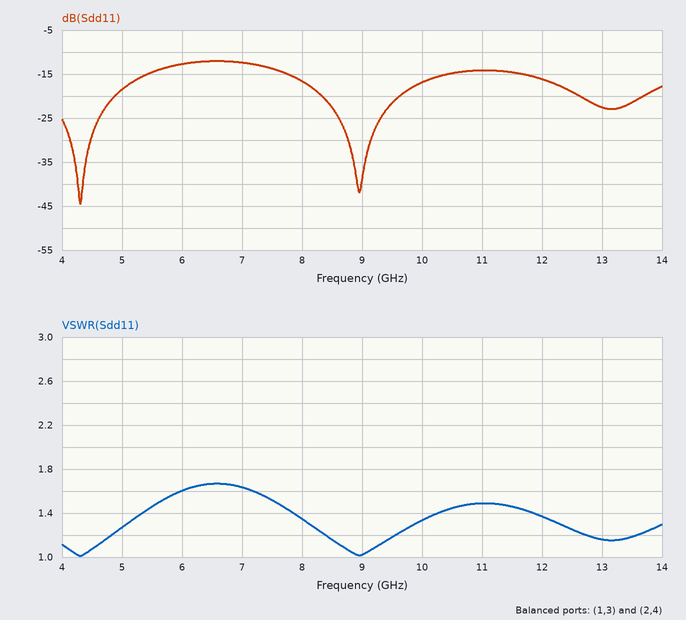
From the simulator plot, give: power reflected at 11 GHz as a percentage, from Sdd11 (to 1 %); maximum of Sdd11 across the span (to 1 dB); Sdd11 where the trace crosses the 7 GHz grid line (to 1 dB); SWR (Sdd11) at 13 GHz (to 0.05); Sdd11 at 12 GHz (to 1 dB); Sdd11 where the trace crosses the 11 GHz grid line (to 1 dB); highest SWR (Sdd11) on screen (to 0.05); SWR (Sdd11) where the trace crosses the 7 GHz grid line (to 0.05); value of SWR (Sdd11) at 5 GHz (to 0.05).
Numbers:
4 %
-12 dB
-12 dB
1.15
-16 dB
-14 dB
1.65
1.65
1.25
